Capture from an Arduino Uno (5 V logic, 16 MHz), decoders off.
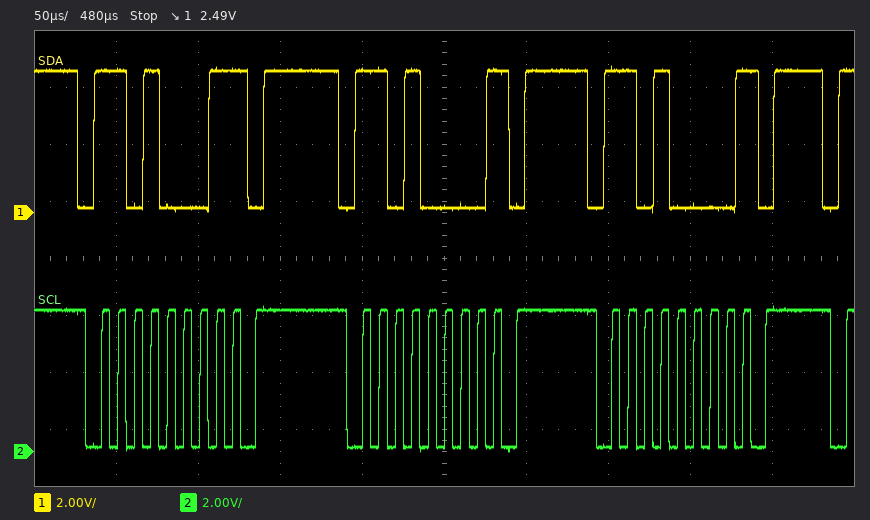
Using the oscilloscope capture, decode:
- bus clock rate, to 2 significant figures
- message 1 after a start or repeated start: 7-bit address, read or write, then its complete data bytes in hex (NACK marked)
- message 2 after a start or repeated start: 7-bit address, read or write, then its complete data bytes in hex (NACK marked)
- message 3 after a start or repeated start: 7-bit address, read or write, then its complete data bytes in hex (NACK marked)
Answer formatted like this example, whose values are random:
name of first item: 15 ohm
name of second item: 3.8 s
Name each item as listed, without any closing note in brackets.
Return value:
bus clock rate, to 2 significant figures: 100 kHz
message 1 after a start or repeated start: 7-bit address, read or write, then its complete data bytes in hex: 0x68 read NACK
message 2 after a start or repeated start: 7-bit address, read or write, then its complete data bytes in hex: 0x68 write NACK
message 3 after a start or repeated start: 7-bit address, read or write, then its complete data bytes in hex: 0x68 write NACK
